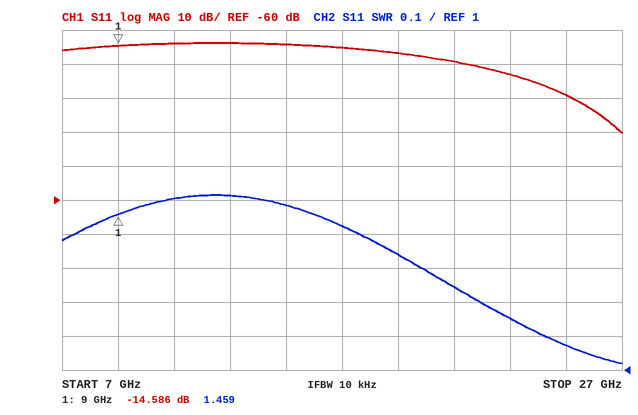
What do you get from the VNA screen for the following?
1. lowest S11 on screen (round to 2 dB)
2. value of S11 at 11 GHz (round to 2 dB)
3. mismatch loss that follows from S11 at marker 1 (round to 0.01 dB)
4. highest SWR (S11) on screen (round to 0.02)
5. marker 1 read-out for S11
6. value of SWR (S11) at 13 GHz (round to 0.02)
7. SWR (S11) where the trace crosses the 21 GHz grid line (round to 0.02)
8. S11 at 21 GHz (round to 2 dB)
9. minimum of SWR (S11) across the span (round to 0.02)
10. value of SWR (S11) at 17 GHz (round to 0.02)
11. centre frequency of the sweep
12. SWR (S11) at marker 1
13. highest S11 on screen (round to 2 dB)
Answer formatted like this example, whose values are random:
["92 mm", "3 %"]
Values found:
["-40 dB", "-14 dB", "0.15 dB", "1.52", "-14.586 dB", "1.52", "1.24", "-20 dB", "1.02", "1.42", "17 GHz", "1.459", "-14 dB"]
